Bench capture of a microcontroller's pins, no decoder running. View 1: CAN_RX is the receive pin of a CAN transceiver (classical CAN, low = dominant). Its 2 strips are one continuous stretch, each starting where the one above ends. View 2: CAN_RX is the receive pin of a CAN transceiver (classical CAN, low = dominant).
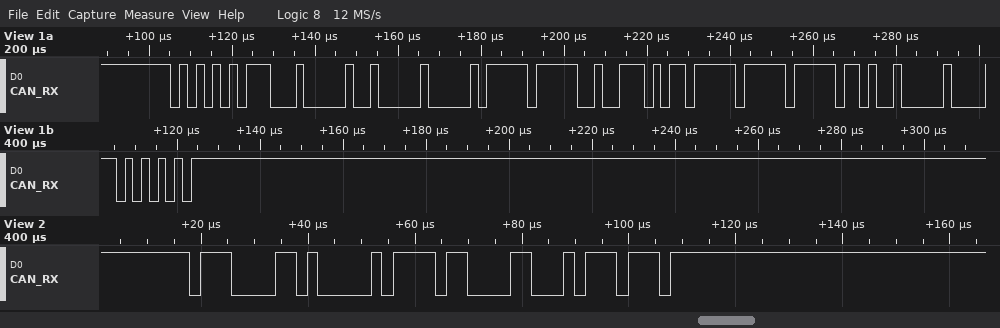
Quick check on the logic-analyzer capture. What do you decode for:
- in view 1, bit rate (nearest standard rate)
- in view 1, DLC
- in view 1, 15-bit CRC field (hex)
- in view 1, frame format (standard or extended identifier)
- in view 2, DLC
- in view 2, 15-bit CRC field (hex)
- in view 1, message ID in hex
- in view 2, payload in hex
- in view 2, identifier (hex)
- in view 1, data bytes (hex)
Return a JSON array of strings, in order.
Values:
["500 kbit/s", "8", "0x01AA", "standard", "1", "0x18BB", "0x557", "EC", "0x70D", "08 00 FF D3 AD FF FF 48"]
